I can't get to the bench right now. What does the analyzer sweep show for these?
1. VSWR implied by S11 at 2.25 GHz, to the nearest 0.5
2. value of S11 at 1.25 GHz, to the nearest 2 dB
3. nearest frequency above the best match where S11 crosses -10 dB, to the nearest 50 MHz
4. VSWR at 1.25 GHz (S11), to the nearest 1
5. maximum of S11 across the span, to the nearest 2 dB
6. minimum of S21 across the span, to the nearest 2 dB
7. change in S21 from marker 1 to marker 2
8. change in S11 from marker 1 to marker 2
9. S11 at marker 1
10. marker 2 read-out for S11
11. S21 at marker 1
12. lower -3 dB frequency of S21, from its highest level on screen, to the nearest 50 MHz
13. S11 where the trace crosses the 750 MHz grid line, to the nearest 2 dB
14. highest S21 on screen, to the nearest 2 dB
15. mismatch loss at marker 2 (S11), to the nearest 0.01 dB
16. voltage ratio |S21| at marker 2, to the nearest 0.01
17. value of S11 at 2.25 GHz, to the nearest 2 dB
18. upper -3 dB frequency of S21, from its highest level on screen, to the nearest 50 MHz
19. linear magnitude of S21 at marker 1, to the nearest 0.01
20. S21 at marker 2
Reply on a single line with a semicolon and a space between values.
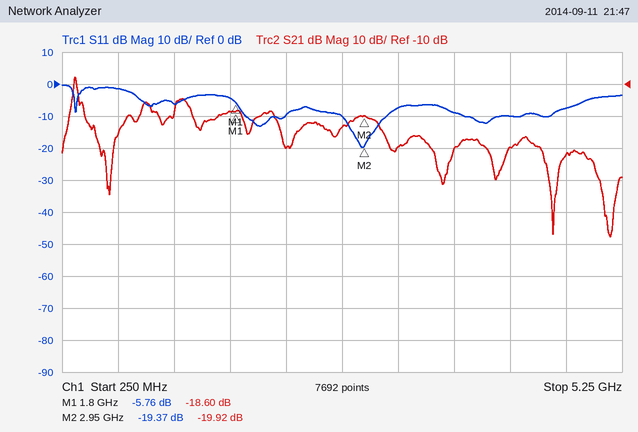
2.0; -6 dB; 3.15 GHz; 3; 0 dB; -58 dB; -1.32 dB; -13.61 dB; -5.76 dB; -19.37 dB; -18.60 dB; 350 MHz; -2 dB; -8 dB; 0.05 dB; 0.10; -10 dB; 400 MHz; 0.12; -19.92 dB
